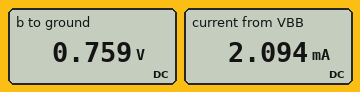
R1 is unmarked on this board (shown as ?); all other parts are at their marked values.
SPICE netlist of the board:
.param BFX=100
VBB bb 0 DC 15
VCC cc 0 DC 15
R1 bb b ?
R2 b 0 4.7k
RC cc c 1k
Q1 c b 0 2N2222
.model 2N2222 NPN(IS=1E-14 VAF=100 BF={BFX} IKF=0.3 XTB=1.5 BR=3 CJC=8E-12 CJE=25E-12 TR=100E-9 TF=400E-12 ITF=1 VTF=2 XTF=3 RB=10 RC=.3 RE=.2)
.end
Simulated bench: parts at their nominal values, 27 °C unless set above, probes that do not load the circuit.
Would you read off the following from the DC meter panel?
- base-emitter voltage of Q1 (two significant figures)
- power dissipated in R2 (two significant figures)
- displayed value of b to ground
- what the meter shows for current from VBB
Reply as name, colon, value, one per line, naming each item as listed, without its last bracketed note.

base-emitter voltage of Q1: 760 mV
power dissipated in R2: 120 µW
displayed value of b to ground: 0.759 V
what the meter shows for current from VBB: 2.094 mA
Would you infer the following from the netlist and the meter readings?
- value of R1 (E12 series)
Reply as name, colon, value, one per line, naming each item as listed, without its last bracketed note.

value of R1: 6.8 kΩ
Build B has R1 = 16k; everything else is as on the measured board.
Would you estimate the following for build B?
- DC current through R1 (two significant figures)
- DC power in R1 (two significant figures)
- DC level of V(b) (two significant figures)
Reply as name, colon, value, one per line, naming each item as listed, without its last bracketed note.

DC current through R1: 890 µA
DC power in R1: 13 mW
DC level of V(b): 740 mV
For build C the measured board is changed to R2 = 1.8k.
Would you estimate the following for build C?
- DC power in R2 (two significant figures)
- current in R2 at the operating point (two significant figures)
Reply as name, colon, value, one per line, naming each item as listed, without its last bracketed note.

DC power in R2: 320 µW
current in R2 at the operating point: 420 µA
